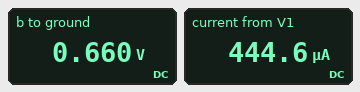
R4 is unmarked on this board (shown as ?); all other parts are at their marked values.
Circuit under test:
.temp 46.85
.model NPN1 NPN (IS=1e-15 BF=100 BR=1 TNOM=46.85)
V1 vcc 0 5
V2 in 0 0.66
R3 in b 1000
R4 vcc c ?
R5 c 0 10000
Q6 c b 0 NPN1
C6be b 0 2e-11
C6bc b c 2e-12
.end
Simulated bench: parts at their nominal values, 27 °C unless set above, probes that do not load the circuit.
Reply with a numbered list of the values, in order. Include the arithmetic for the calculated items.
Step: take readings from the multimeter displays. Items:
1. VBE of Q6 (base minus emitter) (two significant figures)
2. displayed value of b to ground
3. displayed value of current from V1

1. 660 mV = 660 mV
2. 0.660 V
3. 444.6 µA
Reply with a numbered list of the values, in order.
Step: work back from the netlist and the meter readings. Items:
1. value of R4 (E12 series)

1. 1.8 kΩ
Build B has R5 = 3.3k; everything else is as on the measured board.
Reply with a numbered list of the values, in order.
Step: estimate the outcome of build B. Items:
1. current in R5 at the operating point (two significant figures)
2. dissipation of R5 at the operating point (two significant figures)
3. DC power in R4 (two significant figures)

1. 970 µA
2. 3.1 mW
3. 1.8 mW
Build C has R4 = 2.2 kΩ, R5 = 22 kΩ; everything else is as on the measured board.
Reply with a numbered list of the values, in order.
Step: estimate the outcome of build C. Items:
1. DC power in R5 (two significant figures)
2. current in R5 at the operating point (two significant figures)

1. 920 µW
2. 200 µA
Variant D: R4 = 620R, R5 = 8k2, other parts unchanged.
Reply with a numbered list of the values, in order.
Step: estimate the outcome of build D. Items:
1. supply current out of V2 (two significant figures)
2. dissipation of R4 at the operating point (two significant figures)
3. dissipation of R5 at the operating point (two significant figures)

1. 250 nA
2. 220 µW
3. 2.6 mW
